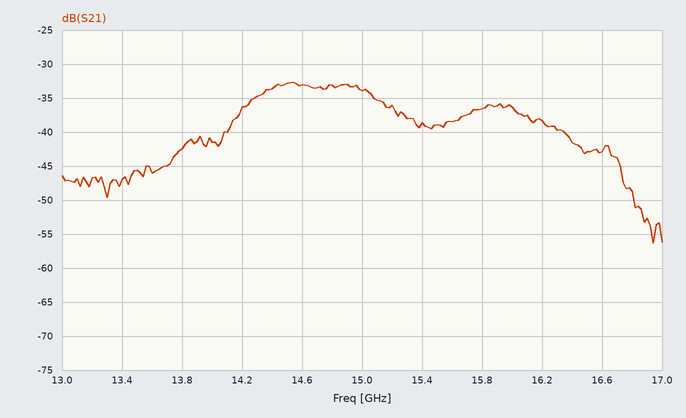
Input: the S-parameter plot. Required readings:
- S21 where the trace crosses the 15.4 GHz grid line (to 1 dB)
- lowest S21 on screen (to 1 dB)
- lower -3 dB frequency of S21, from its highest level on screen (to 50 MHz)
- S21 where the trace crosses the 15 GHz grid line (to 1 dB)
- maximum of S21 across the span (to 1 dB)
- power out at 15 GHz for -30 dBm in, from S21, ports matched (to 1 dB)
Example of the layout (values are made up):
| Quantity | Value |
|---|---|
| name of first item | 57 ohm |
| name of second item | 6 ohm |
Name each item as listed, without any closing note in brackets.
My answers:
| Quantity | Value |
|---|---|
| S21 where the trace crosses the 15.4 GHz grid line | -39 dB |
| lowest S21 on screen | -56 dB |
| lower -3 dB frequency of S21, from its highest level on screen | 14.25 GHz |
| S21 where the trace crosses the 15 GHz grid line | -34 dB |
| maximum of S21 across the span | -33 dB |
| power out at 15 GHz for -30 dBm in, from S21, ports matched | -64 dBm |
